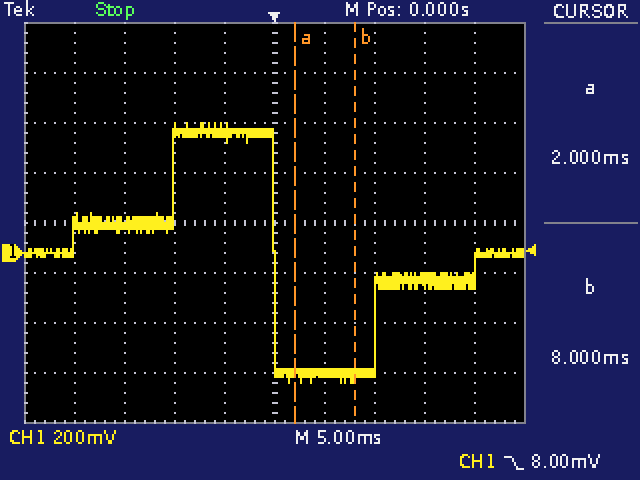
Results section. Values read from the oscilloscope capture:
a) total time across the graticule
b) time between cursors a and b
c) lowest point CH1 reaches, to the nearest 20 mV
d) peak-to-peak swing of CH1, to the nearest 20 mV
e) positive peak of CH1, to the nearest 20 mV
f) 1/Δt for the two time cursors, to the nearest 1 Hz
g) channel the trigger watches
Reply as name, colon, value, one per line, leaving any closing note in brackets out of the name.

total time across the graticule: 50 ms
time between cursors a and b: 6.0 ms
lowest point CH1 reaches, to the nearest 20 mV: -520 mV
peak-to-peak swing of CH1, to the nearest 20 mV: 1.04 V
positive peak of CH1, to the nearest 20 mV: 520 mV
1/Δt for the two time cursors, to the nearest 1 Hz: 167 Hz
channel the trigger watches: CH1
